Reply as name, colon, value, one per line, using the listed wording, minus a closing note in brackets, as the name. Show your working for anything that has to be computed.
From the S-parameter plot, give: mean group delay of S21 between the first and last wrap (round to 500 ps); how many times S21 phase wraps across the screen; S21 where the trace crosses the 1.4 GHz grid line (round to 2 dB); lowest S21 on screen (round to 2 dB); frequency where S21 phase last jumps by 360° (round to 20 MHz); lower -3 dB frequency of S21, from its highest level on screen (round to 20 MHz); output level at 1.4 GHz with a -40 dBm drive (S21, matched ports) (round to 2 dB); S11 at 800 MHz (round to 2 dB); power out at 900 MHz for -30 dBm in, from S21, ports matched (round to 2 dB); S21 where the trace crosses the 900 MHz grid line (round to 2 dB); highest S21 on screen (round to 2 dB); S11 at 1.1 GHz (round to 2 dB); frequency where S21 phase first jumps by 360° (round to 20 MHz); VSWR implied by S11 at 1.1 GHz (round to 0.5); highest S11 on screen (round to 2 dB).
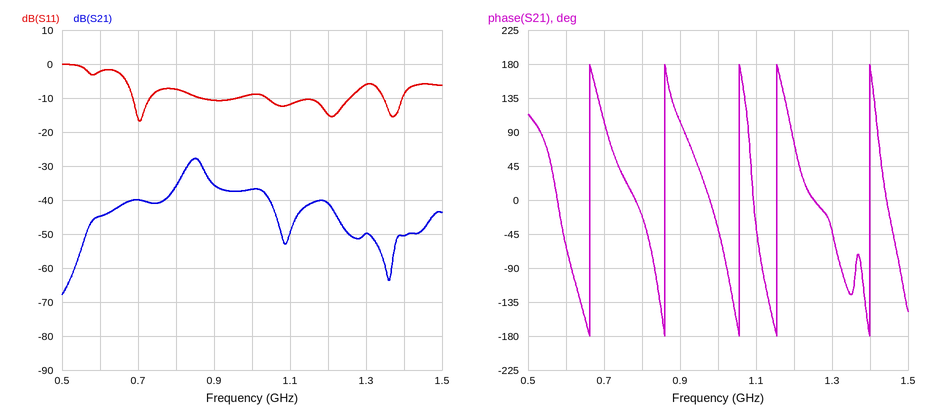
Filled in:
mean group delay of S21 between the first and last wrap: 4 cycles / (1.40 GHz − 660 MHz) ≈ 5.41 ns, so 5.5 ns to the nearest 500 ps
how many times S21 phase wraps across the screen: 5
S21 where the trace crosses the 1.4 GHz grid line: -50 dB
lowest S21 on screen: -68 dB
frequency where S21 phase last jumps by 360°: 1.40 GHz
lower -3 dB frequency of S21, from its highest level on screen: 820 MHz
output level at 1.4 GHz with a -40 dBm drive (S21, matched ports): -40 dBm + (-50 dB) = -90 dBm
S11 at 800 MHz: -8 dB
power out at 900 MHz for -30 dBm in, from S21, ports matched: -30 dBm + (-36 dB) = -66 dBm
S21 where the trace crosses the 900 MHz grid line: -36 dB
highest S21 on screen: -28 dB
S11 at 1.1 GHz: -12 dB
frequency where S21 phase first jumps by 360°: 660 MHz
VSWR implied by S11 at 1.1 GHz: |Γ| = 10^(-12/20) = 0.2512; VSWR = (1 + 0.2512)/(1 − 0.2512) ≈ 1.67, so 1.5 to the nearest 0.5
highest S11 on screen: 0 dB
